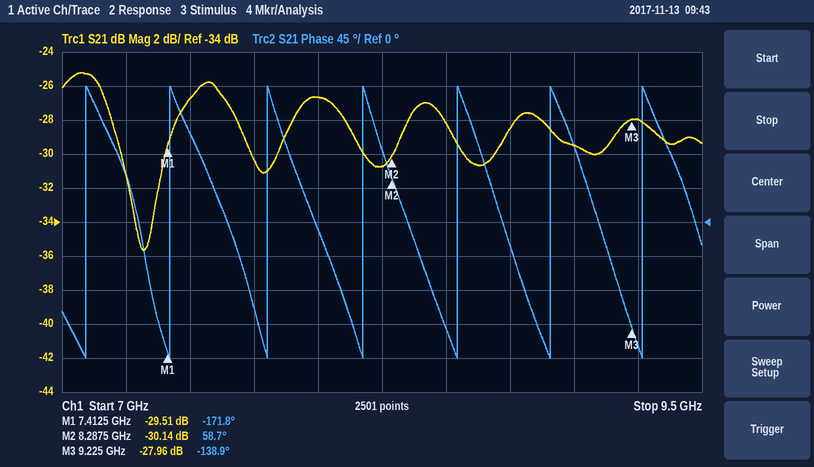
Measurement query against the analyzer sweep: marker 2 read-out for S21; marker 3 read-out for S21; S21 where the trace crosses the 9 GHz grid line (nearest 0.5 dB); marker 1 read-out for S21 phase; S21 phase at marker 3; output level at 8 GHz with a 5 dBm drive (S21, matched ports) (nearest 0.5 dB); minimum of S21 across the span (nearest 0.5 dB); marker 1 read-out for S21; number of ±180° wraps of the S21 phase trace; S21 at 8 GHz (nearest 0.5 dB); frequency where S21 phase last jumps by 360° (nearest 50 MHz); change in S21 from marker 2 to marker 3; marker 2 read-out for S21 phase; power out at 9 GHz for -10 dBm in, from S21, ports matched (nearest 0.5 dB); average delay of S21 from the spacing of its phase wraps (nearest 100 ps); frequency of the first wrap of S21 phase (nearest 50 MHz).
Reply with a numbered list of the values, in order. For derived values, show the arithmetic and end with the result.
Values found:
1. -30.14 dB
2. -27.96 dB
3. -29.5 dB
4. -171.8°
5. -138.9°
6. 5 dBm + (-26.5 dB) = -21.5 dBm
7. -35.5 dB
8. -29.51 dB
9. 7
10. -26.5 dB
11. 9.25 GHz
12. -27.96 − (-30.14) = 2.18 dB
13. 58.7°
14. -10 dBm + (-29.5 dB) = -39.5 dBm
15. 6 cycles / (9.25 GHz − 7.10 GHz) ≈ 2.8 ns
16. 7.10 GHz
